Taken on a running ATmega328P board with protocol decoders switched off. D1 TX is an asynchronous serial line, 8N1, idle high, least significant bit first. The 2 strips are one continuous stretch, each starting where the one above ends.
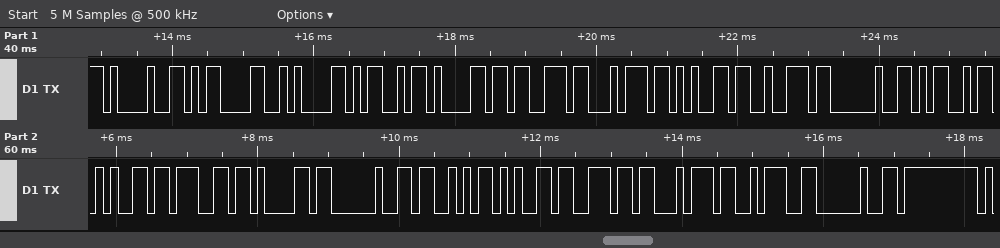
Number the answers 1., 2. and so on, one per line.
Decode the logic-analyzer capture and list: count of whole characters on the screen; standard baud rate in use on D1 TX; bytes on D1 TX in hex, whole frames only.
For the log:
1. 22
2. 9600 baud
3. 21 0D 0A 4D 61 73 74 65 72 20 4D 65 67 61 20 53 65 6E 74 3A 20 FF
